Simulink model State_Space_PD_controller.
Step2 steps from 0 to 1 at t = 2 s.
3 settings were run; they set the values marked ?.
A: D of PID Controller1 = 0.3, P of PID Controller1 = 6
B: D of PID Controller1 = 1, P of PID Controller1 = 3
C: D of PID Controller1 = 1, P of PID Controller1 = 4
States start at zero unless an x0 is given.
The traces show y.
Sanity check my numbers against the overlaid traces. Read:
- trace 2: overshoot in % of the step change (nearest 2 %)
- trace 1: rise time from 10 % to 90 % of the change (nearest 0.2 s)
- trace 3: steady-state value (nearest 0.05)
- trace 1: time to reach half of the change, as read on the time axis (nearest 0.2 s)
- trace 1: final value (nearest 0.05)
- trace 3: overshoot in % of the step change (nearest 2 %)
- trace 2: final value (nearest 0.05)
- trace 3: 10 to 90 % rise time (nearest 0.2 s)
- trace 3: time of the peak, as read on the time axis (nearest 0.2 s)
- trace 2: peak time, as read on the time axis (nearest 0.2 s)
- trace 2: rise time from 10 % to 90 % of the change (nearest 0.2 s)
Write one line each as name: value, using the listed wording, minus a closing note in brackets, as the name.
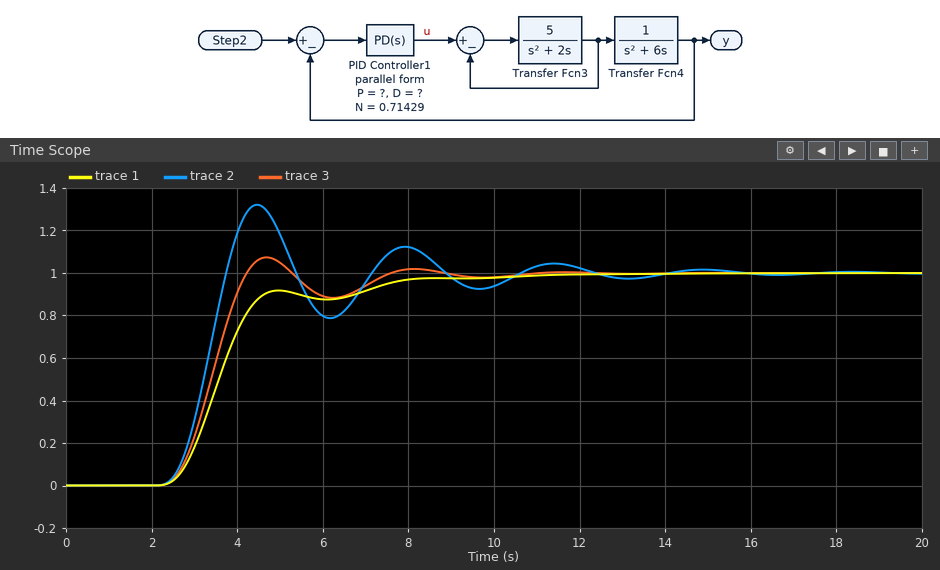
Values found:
trace 2: overshoot in % of the step change: 32 %
trace 1: rise time from 10 % to 90 % of the change: 1.8 s
trace 3: steady-state value: 1.00
trace 1: time to reach half of the change, as read on the time axis: 3.6 s
trace 1: final value: 1.00
trace 3: overshoot in % of the step change: 8 %
trace 2: final value: 1.00
trace 3: 10 to 90 % rise time: 1.2 s
trace 3: time of the peak, as read on the time axis: 4.6 s
trace 2: peak time, as read on the time axis: 4.4 s
trace 2: rise time from 10 % to 90 % of the change: 1.0 s
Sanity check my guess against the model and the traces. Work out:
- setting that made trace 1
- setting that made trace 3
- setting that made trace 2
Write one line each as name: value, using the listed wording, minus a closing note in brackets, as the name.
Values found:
setting that made trace 1: B
setting that made trace 3: C
setting that made trace 2: A
